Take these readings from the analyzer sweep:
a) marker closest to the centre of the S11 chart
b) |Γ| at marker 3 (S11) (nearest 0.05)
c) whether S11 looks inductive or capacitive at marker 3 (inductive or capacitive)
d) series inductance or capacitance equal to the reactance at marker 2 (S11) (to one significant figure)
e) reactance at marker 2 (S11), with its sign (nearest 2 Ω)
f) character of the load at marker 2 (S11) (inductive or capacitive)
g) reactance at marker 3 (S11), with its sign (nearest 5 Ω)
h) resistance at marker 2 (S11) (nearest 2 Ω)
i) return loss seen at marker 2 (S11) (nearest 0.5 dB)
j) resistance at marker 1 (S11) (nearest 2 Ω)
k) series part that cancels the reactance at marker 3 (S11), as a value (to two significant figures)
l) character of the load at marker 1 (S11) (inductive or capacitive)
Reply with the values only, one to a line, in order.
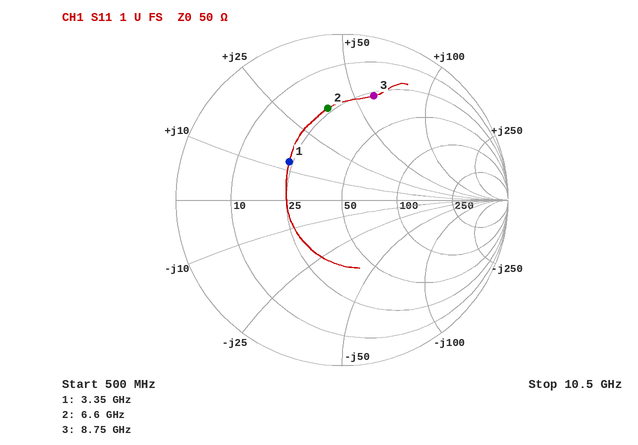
marker 1
0.65
inductive
900 pH
+38 Ω
inductive
+60 Ω
24 Ω
5.0 dB
24 Ω
300 fF
inductive
